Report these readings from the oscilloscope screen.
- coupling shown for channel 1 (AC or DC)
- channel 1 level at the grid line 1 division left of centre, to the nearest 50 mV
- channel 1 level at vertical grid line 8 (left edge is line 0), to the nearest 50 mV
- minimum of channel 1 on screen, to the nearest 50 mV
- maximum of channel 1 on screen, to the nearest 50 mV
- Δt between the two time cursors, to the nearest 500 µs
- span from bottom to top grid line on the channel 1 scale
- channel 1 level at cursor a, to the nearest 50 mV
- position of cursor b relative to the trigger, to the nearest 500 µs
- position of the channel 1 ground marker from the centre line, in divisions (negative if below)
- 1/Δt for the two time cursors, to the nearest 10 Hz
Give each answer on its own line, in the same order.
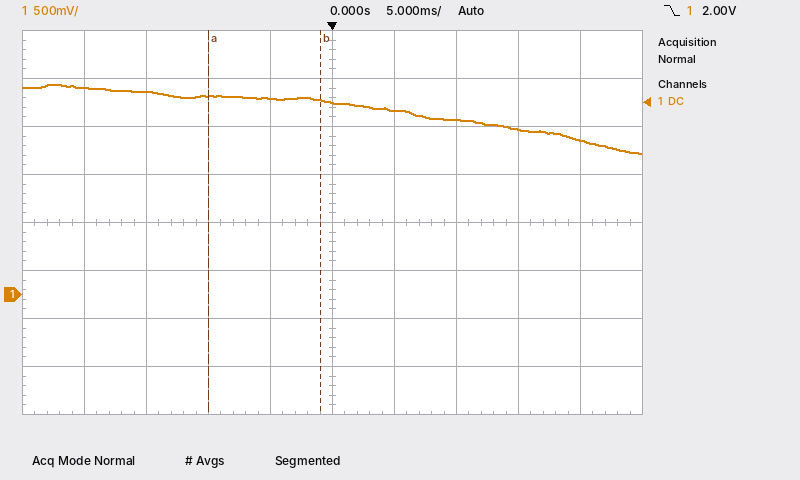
DC
2.05 V
1.70 V
1.45 V
2.20 V
9.0 ms
4 V
2.05 V
-1.0 ms
-1.5 div
110 Hz
